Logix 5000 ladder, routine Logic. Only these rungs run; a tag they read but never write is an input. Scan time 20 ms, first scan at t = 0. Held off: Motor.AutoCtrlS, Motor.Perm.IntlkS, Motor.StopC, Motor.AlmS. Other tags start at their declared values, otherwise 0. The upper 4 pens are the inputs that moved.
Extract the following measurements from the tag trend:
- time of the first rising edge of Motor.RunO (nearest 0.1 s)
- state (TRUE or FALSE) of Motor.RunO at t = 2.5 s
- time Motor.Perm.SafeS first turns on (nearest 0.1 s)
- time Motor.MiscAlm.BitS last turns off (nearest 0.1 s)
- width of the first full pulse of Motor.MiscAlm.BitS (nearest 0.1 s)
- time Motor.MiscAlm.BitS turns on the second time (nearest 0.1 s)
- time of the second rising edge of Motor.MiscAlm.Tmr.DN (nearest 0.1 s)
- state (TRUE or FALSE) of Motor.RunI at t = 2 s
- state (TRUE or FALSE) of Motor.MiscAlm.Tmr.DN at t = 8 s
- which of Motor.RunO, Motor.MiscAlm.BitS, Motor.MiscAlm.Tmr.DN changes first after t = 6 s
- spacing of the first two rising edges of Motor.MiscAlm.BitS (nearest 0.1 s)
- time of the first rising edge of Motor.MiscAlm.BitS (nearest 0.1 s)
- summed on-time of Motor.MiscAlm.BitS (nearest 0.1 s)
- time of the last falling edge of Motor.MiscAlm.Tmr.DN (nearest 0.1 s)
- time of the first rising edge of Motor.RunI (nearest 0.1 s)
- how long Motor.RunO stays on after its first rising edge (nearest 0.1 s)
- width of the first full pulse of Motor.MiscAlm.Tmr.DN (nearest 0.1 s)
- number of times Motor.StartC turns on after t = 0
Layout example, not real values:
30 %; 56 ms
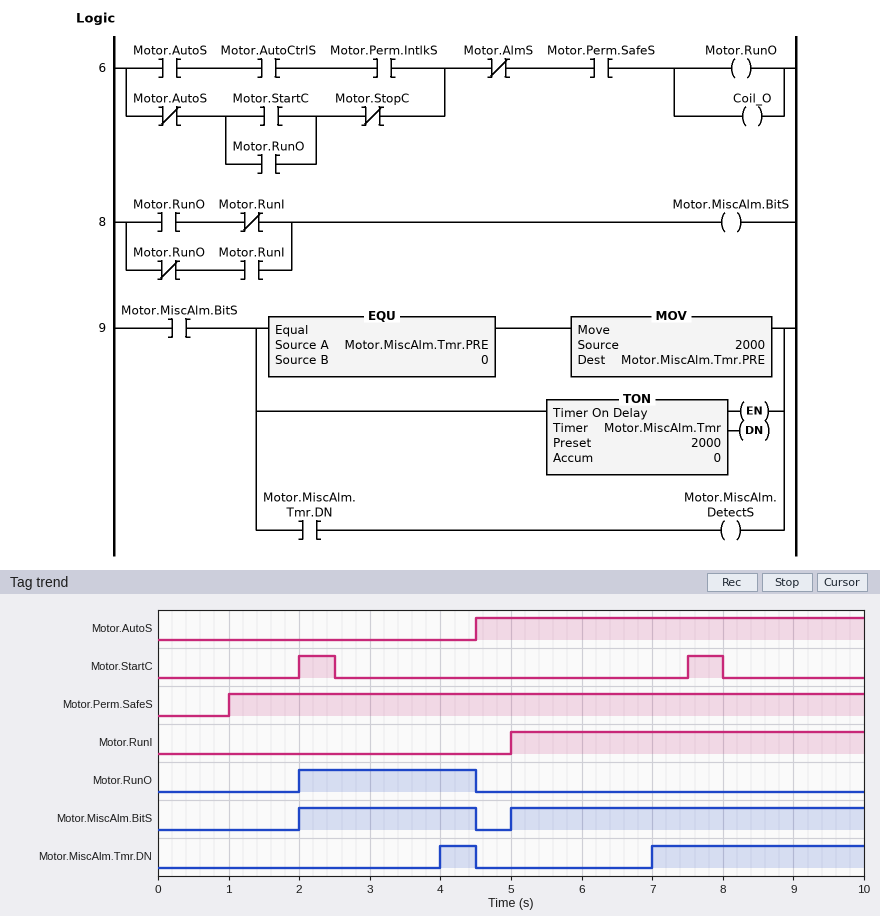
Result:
2.0 s; TRUE; 1.0 s; 4.5 s; 2.5 s; 5.0 s; 7.0 s; FALSE; TRUE; Motor.MiscAlm.Tmr.DN; 3.0 s; 2.0 s; 7.5 s; 4.5 s; 5.0 s; 2.5 s; 0.5 s; 2
